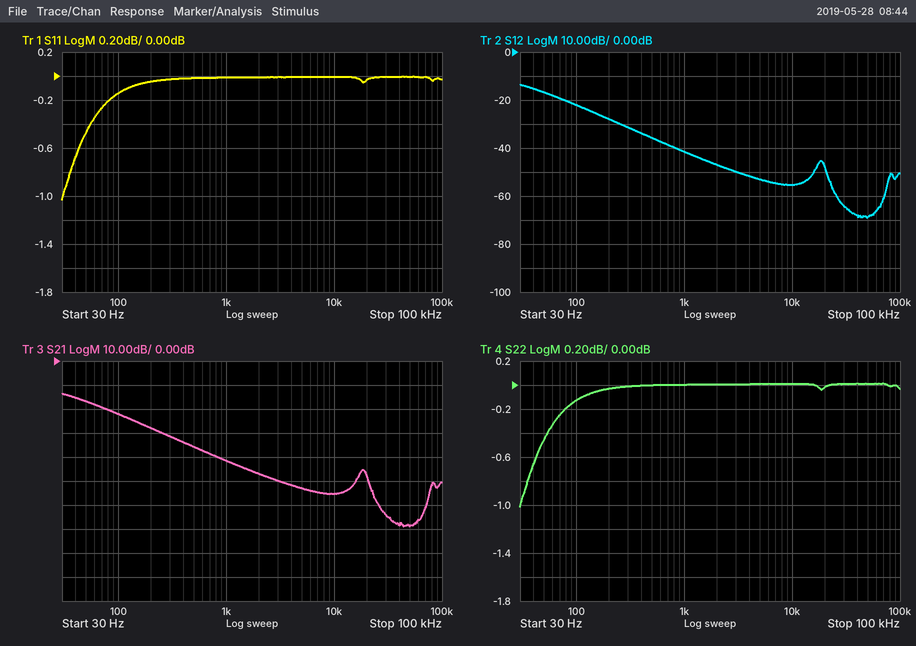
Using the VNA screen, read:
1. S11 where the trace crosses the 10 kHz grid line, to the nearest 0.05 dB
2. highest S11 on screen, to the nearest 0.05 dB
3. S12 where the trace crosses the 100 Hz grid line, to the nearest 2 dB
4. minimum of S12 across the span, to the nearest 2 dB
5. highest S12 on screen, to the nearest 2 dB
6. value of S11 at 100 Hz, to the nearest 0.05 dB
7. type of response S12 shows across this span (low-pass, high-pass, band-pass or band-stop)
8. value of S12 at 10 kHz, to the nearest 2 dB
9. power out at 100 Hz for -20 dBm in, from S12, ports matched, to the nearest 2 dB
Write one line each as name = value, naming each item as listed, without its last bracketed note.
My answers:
S11 where the trace crosses the 10 kHz grid line, to the nearest 0.05 dB = 0.00 dB
highest S11 on screen, to the nearest 0.05 dB = 0.00 dB
S12 where the trace crosses the 100 Hz grid line, to the nearest 2 dB = -22 dB
minimum of S12 across the span, to the nearest 2 dB = -70 dB
highest S12 on screen, to the nearest 2 dB = -14 dB
value of S11 at 100 Hz, to the nearest 0.05 dB = -0.15 dB
type of response S12 shows across this span = low-pass
value of S12 at 10 kHz, to the nearest 2 dB = -56 dB
power out at 100 Hz for -20 dBm in, from S12, ports matched, to the nearest 2 dB = -42 dBm
